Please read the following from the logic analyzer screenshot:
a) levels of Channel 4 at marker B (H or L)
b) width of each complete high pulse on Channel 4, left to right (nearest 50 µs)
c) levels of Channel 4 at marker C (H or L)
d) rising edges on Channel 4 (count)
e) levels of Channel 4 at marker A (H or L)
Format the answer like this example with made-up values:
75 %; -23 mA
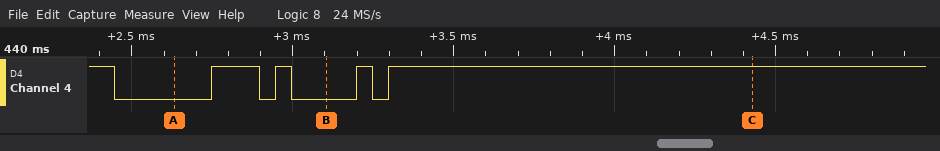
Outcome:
Channel 4=L; 150 µs, 50 µs, 50 µs; Channel 4=H; 4; Channel 4=L
